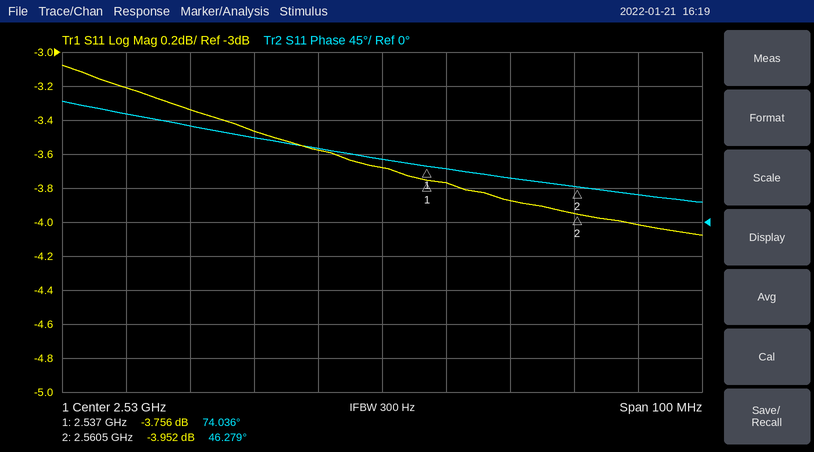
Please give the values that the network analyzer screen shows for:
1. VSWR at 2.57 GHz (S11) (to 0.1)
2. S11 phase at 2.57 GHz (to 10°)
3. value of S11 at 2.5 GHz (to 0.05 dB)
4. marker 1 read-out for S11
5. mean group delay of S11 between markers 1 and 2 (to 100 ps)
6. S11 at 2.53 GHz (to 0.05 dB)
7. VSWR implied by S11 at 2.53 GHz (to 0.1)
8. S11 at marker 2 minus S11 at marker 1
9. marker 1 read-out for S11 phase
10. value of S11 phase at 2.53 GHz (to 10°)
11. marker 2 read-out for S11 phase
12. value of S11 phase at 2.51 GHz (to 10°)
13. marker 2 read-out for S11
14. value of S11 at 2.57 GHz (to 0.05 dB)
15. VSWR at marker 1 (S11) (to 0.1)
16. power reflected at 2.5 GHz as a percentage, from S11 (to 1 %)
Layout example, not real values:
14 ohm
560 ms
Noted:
4.4
40°
-3.35 dB
-3.756 dB
3.3 ns
-3.70 dB
4.8
-0.196 dB
74.036°
80°
46.279°
110°
-3.952 dB
-4.00 dB
4.7
46 %
